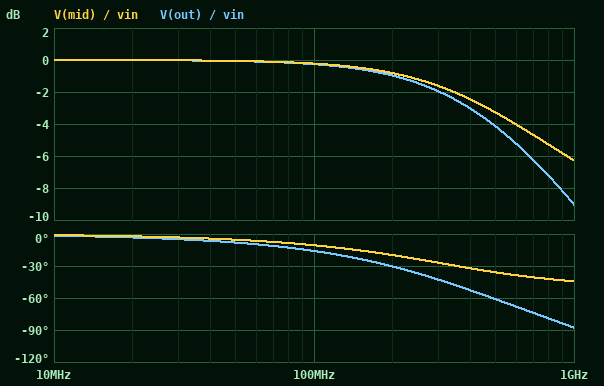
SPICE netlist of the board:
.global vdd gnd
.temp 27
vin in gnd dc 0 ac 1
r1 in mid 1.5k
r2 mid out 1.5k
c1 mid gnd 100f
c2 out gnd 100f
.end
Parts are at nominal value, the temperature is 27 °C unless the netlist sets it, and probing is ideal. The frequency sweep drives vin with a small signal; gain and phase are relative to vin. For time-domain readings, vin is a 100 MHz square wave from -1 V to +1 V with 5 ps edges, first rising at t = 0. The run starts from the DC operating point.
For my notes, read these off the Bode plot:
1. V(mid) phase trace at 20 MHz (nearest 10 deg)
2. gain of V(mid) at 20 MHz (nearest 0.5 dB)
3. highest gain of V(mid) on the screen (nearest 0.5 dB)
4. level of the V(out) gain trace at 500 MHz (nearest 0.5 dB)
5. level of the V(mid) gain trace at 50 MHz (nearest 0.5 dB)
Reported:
0 deg
0 dB
0 dB
-4.0 dB
0 dB
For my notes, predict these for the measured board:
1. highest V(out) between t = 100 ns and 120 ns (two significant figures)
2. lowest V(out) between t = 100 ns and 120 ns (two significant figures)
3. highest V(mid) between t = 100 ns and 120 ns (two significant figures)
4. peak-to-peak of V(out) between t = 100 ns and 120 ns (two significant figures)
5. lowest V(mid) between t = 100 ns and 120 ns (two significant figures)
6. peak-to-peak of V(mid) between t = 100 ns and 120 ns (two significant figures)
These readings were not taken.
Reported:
1.0 V
-1.0 V
1.0 V
2.0 V
-1.0 V
2.0 V
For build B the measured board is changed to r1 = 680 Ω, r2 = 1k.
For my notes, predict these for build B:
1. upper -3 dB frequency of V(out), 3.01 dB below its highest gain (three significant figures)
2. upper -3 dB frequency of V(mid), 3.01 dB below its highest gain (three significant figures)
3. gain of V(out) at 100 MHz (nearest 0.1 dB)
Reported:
766 MHz
1.03 GHz
-0.1 dB
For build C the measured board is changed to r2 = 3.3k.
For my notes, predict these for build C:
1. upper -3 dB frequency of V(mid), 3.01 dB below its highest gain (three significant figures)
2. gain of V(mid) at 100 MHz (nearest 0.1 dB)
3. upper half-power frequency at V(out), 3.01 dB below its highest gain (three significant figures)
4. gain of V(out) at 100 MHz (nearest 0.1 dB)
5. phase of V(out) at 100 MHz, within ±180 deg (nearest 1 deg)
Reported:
494 MHz
-0.3 dB
288 MHz
-0.5 dB
-22 deg
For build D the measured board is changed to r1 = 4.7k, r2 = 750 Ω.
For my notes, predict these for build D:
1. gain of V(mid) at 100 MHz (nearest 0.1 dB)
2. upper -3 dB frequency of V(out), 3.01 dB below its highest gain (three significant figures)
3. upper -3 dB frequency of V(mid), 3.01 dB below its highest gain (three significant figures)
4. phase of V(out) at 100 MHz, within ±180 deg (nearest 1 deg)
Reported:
-1.4 dB
162 MHz
163 MHz
-33 deg
